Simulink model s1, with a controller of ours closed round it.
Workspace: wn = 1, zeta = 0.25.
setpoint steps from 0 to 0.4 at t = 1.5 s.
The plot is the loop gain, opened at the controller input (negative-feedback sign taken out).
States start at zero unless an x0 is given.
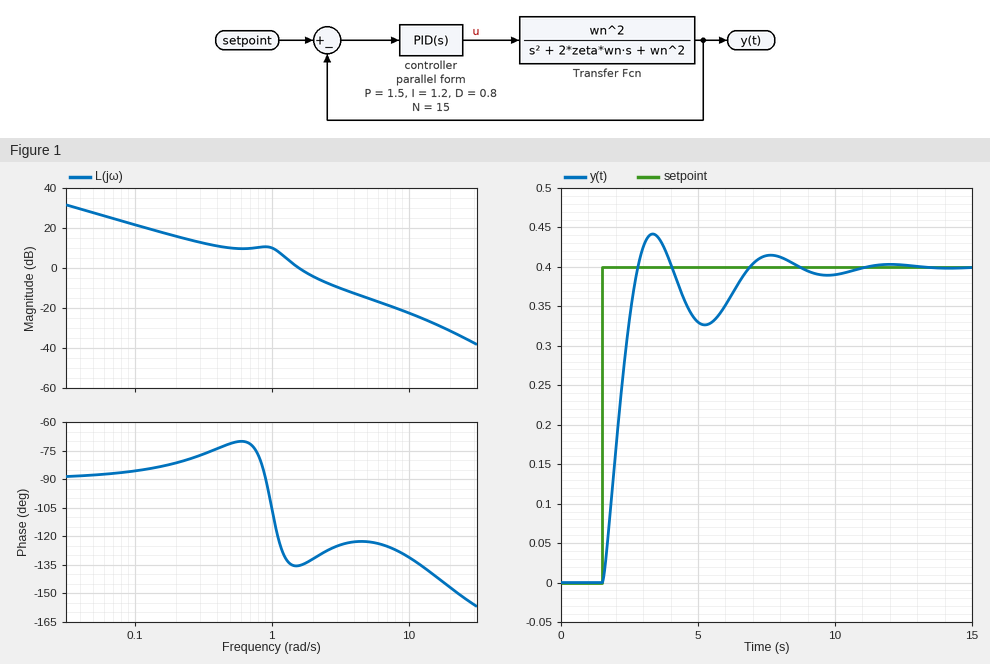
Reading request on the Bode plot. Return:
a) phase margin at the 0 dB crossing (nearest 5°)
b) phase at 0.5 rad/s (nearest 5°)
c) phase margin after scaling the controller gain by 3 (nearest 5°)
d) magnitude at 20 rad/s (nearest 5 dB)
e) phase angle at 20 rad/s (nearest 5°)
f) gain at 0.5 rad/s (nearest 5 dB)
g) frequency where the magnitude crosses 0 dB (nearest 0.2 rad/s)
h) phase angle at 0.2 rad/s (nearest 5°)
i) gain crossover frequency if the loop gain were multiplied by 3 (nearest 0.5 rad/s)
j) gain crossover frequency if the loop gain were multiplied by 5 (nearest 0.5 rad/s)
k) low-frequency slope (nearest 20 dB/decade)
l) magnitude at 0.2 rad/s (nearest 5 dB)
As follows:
45°
-70°
55°
-30 dB
-145°
10 dB
1.6 rad/s
-80°
3.0 rad/s
4.5 rad/s
-20 dB/decade
15 dB
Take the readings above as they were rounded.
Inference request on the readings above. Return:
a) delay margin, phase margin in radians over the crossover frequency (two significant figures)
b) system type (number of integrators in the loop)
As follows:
0.49 s
1
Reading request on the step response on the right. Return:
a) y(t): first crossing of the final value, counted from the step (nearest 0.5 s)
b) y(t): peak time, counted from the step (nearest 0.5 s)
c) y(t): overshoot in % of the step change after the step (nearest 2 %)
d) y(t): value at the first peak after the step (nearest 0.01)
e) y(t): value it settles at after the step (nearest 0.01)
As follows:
1.5 s
2.0 s
10 %
0.44
0.40
